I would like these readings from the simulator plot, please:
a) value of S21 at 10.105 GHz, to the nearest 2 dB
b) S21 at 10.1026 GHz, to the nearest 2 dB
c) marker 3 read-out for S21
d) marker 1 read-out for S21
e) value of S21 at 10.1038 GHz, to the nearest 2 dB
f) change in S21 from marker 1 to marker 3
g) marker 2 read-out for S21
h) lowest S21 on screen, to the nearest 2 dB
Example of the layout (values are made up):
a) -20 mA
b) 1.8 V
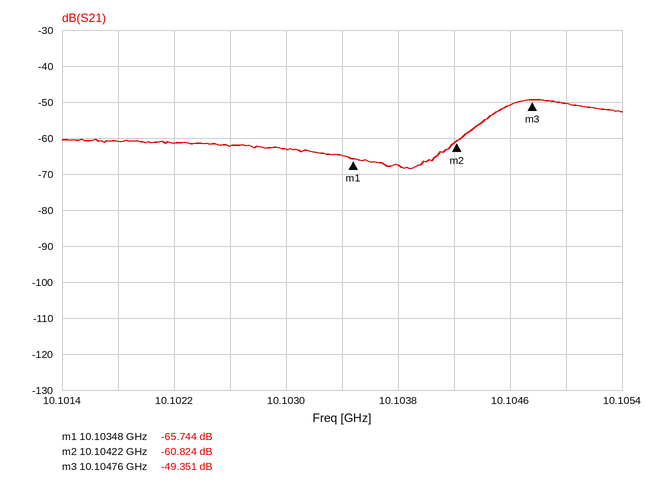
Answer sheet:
a) -50 dB
b) -62 dB
c) -49.351 dB
d) -65.744 dB
e) -68 dB
f) 16.393 dB
g) -60.824 dB
h) -68 dB
